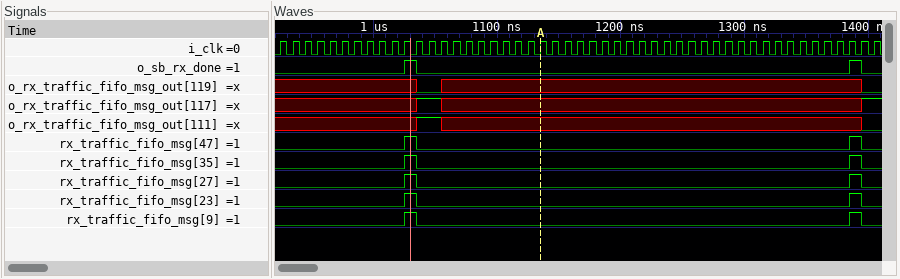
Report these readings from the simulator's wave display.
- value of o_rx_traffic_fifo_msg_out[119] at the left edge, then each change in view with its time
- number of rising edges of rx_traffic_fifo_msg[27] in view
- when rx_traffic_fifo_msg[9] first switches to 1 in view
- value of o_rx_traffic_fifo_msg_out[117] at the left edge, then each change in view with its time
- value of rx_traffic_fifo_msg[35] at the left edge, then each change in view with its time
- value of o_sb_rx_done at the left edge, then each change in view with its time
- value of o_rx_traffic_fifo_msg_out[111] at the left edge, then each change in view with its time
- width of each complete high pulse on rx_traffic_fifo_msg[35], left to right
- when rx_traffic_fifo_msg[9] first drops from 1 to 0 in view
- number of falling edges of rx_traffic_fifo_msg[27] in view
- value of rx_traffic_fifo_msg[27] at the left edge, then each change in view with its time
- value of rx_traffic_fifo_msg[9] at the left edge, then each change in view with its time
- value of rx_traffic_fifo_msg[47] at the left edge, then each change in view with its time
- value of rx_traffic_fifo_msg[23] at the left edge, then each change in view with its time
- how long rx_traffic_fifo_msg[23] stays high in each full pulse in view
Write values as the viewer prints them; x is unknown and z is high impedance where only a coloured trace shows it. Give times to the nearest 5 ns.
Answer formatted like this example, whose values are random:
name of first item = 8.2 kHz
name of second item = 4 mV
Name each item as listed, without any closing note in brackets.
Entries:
value of o_rx_traffic_fifo_msg_out[119] at the left edge, then each change in view with its time = x, 0 at 1035 ns, x at 1055 ns, 0 at 1395 ns
number of rising edges of rx_traffic_fifo_msg[27] in view = 2
when rx_traffic_fifo_msg[9] first switches to 1 in view = 1025 ns
value of o_rx_traffic_fifo_msg_out[117] at the left edge, then each change in view with its time = x, 1 at 1035 ns, x at 1055 ns, 1 at 1395 ns
value of rx_traffic_fifo_msg[35] at the left edge, then each change in view with its time = 0, 1 at 1025 ns, 0 at 1035 ns, 1 at 1385 ns, 0 at 1395 ns
value of o_sb_rx_done at the left edge, then each change in view with its time = 0, 1 at 1025 ns, 0 at 1035 ns, 1 at 1385 ns, 0 at 1395 ns
value of o_rx_traffic_fifo_msg_out[111] at the left edge, then each change in view with its time = x, 1 at 1035 ns, x at 1055 ns, 0 at 1395 ns
width of each complete high pulse on rx_traffic_fifo_msg[35], left to right = 10 ns, 10 ns
when rx_traffic_fifo_msg[9] first drops from 1 to 0 in view = 1035 ns
number of falling edges of rx_traffic_fifo_msg[27] in view = 2
value of rx_traffic_fifo_msg[27] at the left edge, then each change in view with its time = 0, 1 at 1025 ns, 0 at 1035 ns, 1 at 1385 ns, 0 at 1395 ns
value of rx_traffic_fifo_msg[9] at the left edge, then each change in view with its time = 0, 1 at 1025 ns, 0 at 1035 ns, 1 at 1385 ns, 0 at 1395 ns
value of rx_traffic_fifo_msg[47] at the left edge, then each change in view with its time = 0, 1 at 1025 ns, 0 at 1035 ns, 1 at 1385 ns, 0 at 1395 ns
value of rx_traffic_fifo_msg[23] at the left edge, then each change in view with its time = 0, 1 at 1025 ns, 0 at 1035 ns, 1 at 1385 ns, 0 at 1395 ns
how long rx_traffic_fifo_msg[23] stays high in each full pulse in view = 10 ns, 10 ns
